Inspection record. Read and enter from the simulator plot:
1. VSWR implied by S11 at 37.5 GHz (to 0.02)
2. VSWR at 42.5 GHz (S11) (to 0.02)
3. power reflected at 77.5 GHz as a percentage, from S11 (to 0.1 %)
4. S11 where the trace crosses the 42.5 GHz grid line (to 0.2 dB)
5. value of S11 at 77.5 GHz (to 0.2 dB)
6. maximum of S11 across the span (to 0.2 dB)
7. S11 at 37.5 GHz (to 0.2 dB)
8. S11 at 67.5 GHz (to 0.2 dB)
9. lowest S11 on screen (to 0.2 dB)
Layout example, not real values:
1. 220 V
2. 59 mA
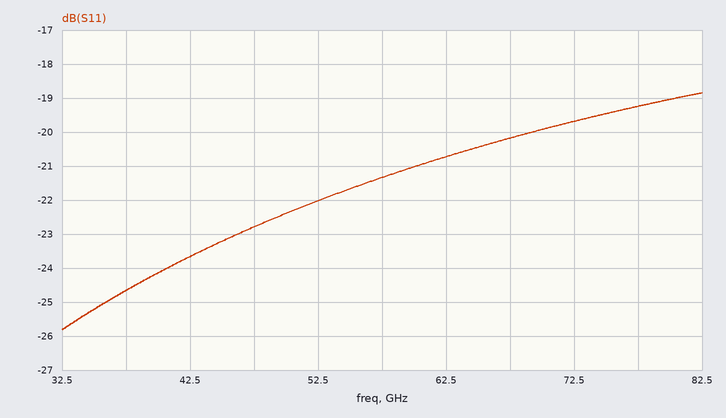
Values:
1. 1.12
2. 1.14
3. 1.2 %
4. -23.6 dB
5. -19.2 dB
6. -18.8 dB
7. -24.6 dB
8. -20.2 dB
9. -25.8 dB
